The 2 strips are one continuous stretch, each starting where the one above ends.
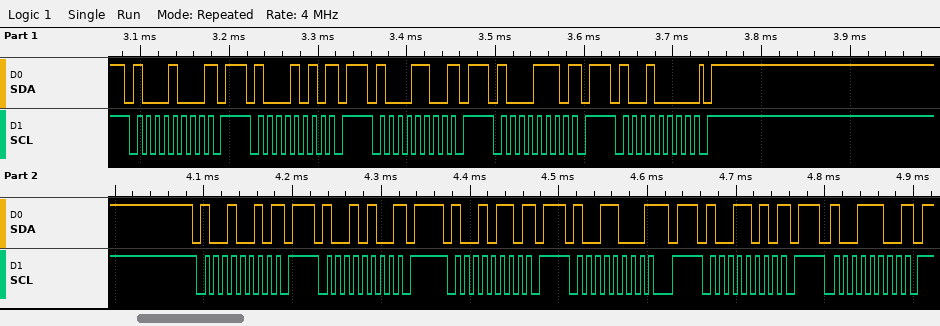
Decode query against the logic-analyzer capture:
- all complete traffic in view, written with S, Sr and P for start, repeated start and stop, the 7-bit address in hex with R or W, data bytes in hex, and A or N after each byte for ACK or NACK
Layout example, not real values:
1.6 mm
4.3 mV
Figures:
S 44W N P S 45W N P S 46W N P S 47W N P S 48W A P S 49W N P S 4AW N P S 4BW N P S 4CW N P S 4DW N P S 4EW N P
